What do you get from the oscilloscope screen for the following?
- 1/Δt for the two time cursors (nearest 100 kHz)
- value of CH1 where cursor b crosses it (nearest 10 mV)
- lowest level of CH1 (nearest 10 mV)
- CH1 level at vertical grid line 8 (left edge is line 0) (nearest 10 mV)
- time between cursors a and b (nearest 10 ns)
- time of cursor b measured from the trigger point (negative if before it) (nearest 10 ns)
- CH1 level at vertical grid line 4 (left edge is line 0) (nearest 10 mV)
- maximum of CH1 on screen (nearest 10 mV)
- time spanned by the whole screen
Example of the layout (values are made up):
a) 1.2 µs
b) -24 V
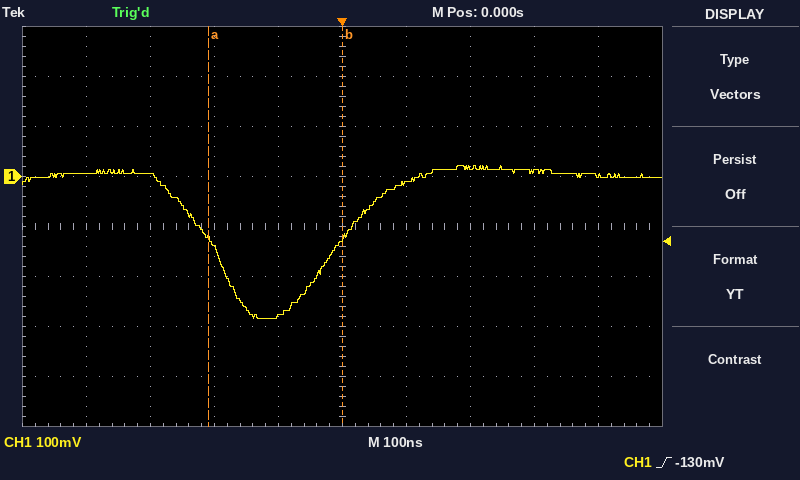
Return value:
a) 4.8 MHz
b) -120 mV
c) -280 mV
d) 10 mV
e) 210 ns
f) 0 ns
g) -280 mV
h) 20 mV
i) 1 µs
